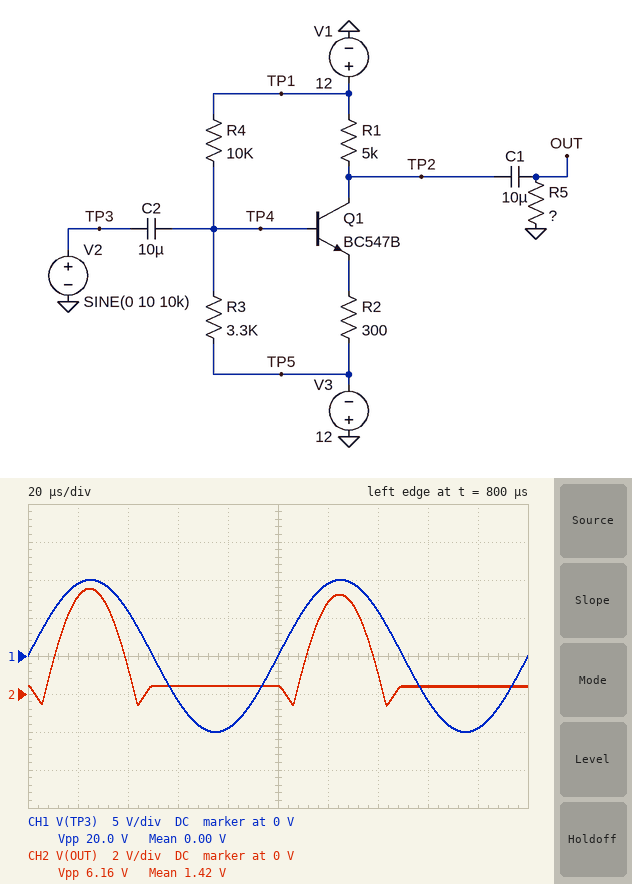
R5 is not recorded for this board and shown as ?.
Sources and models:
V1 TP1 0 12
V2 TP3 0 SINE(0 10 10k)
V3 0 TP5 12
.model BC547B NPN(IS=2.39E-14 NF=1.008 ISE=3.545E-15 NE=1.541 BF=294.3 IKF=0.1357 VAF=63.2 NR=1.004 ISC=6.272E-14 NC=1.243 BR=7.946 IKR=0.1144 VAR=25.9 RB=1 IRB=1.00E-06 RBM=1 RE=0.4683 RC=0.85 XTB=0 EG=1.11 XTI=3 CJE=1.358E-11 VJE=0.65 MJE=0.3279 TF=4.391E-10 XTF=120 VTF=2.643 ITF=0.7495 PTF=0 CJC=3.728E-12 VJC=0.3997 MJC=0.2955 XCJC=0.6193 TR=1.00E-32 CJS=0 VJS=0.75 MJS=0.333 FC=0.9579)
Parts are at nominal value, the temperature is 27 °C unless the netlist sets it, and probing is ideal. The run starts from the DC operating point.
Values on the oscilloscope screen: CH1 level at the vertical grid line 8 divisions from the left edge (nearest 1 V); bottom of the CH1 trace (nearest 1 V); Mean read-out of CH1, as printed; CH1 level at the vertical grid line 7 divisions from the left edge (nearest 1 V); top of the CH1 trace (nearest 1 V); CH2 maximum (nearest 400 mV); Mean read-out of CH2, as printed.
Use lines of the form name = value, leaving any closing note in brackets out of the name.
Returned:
CH1 level at the vertical grid line 8 divisions from the left edge = -6 V
bottom of the CH1 trace = -10 V
Mean read-out of CH1, as printed = 0.00 V
CH1 level at the vertical grid line 7 divisions from the left edge = 6 V
top of the CH1 trace = 10 V
CH2 maximum = 5.6 V
Mean read-out of CH2, as printed = 1.42 V
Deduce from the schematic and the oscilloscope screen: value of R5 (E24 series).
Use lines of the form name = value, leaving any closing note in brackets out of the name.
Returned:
value of R5 = 100 Ω
